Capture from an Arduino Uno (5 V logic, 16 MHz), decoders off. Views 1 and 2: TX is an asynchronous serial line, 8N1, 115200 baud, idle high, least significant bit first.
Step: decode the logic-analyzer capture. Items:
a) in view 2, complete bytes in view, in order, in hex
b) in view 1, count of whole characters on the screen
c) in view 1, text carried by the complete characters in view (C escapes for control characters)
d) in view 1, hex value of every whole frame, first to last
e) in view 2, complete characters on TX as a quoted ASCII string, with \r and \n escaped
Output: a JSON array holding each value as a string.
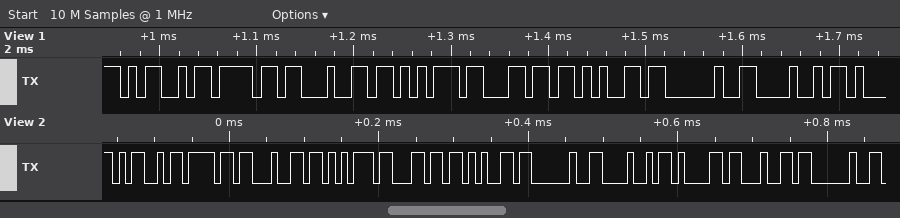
["4D 6F 64 75 6C 65 20 48 61 64 20", "8", "\"Module H\"", "4D 6F 64 75 6C 65 20 48", "\"Module Had \""]
